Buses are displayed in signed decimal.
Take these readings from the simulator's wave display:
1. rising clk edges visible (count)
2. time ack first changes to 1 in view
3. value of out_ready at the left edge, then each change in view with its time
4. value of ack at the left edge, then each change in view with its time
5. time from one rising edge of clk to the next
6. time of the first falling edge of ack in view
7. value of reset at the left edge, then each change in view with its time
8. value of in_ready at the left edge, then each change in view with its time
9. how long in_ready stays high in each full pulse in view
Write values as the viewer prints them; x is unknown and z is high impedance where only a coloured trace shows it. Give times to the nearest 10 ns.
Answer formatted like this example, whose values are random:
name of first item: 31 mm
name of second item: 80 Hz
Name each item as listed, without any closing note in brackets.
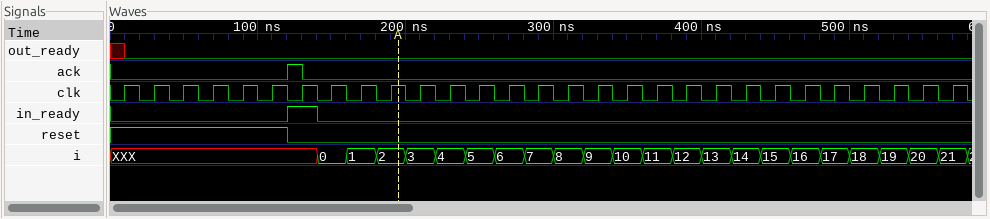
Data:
rising clk edges visible: 29
time ack first changes to 1 in view: 120 ns
value of out_ready at the left edge, then each change in view with its time: x, 0 at 10 ns
value of ack at the left edge, then each change in view with its time: 0, 1 at 120 ns, 0 at 130 ns
time from one rising edge of clk to the next: 20 ns
time of the first falling edge of ack in view: 130 ns
value of reset at the left edge, then each change in view with its time: 1, 0 at 120 ns
value of in_ready at the left edge, then each change in view with its time: 0, 1 at 120 ns, 0 at 140 ns
how long in_ready stays high in each full pulse in view: 20 ns
